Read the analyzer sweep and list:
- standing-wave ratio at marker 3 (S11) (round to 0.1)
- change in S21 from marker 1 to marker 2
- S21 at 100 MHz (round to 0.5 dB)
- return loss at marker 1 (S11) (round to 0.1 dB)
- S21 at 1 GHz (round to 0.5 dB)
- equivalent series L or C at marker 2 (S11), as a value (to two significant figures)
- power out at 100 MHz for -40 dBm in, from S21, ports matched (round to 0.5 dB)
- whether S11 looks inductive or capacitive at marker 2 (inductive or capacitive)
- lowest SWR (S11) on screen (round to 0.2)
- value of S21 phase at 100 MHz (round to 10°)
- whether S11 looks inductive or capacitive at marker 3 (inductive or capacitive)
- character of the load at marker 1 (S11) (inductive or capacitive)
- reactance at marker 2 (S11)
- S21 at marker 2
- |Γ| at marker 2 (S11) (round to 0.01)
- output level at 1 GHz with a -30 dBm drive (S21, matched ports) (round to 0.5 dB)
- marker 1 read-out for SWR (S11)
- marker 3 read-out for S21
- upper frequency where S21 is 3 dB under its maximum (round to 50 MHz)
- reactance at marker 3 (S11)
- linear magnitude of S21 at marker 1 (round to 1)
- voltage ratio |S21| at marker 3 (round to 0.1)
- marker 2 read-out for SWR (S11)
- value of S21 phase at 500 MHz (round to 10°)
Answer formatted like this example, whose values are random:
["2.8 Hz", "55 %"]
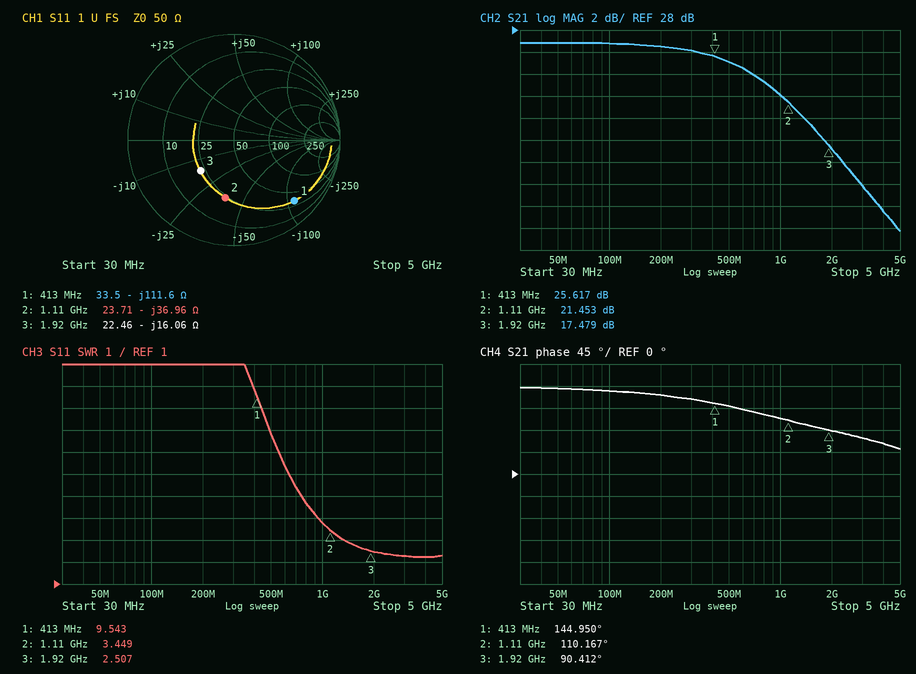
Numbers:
["2.5", "-4.164 dB", "27.0 dB", "1.8 dB", "22.0 dB", "3.9 pF", "-13.0 dBm", "capacitive", "2.2", "170°", "capacitive", "capacitive", "-36.96 Ω", "21.453 dB", "0.55", "-8.0 dBm", "9.543", "17.479 dB", "700 MHz", "-16.06 Ω", "19", "7.5", "3.449", "140°"]
